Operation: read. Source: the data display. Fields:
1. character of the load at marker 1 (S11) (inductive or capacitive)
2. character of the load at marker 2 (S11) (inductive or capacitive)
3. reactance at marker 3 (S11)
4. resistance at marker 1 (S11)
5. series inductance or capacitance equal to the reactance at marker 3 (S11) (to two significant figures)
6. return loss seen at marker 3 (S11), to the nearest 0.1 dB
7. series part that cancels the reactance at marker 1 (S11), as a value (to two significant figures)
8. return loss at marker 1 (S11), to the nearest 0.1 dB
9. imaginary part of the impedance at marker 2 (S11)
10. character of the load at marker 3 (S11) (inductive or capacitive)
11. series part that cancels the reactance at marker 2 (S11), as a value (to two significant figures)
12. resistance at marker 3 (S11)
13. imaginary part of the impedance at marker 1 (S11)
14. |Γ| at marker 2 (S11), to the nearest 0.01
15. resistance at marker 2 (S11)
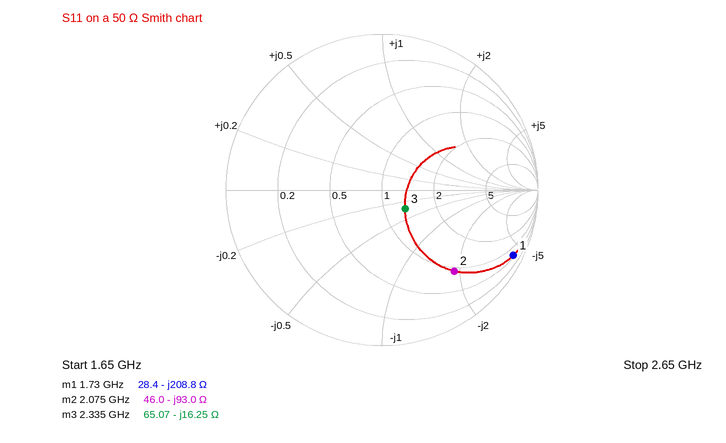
capacitive
capacitive
-16.25 Ω
28.4 Ω
4.2 pF
14.4 dB
19 nH
0.5 dB
-93.0 Ω
capacitive
7.1 nH
65.07 Ω
-208.8 Ω
0.70
46.0 Ω
